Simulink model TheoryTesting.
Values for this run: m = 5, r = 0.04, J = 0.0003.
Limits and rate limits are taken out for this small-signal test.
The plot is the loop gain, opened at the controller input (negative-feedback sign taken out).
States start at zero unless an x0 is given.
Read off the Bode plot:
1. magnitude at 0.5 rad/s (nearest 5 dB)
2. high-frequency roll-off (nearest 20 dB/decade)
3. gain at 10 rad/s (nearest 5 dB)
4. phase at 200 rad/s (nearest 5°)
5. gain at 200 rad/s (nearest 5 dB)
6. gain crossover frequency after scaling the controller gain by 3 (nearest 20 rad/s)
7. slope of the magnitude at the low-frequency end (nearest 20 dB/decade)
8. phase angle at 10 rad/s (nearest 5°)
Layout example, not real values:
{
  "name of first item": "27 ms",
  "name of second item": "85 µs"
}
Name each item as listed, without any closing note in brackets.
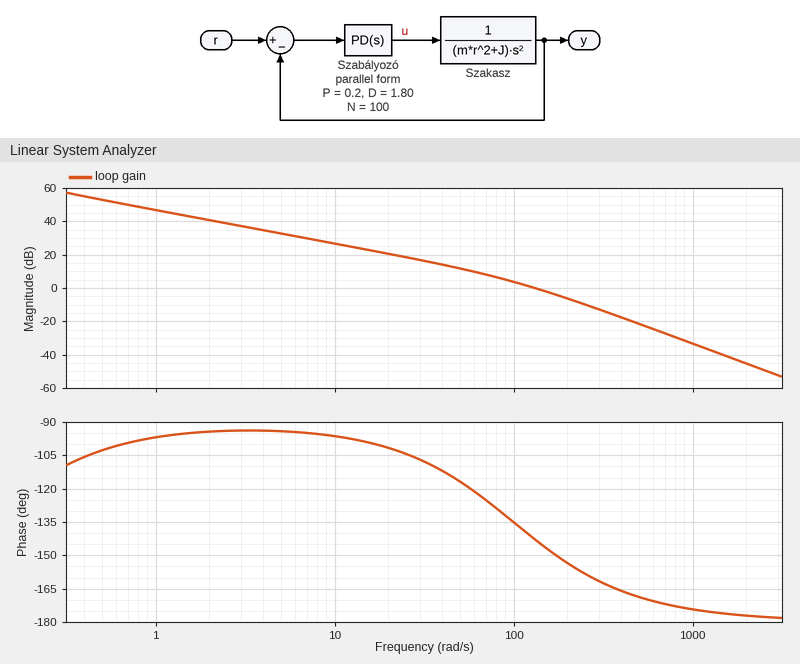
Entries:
{
  "magnitude at 0.5 rad/s": "55 dB",
  "high-frequency roll-off": "-40 dB/decade",
  "gain at 10 rad/s": "25 dB",
  "phase at 200 rad/s": "-155°",
  "gain at 200 rad/s": "-5 dB",
  "gain crossover frequency after scaling the controller gain by 3": "240 rad/s",
  "slope of the magnitude at the low-frequency end": "-20 dB/decade",
  "phase angle at 10 rad/s": "-95°"
}
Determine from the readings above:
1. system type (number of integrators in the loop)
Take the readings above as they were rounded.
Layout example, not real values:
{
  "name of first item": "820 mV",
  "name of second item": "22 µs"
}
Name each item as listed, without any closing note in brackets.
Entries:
{
  "system type": "1"
}
